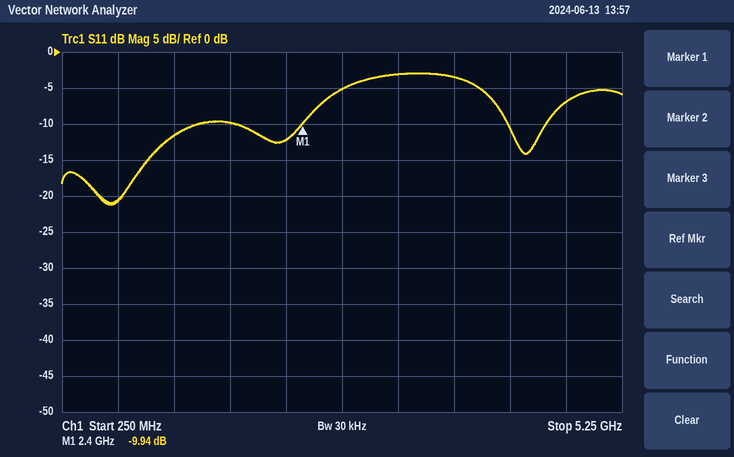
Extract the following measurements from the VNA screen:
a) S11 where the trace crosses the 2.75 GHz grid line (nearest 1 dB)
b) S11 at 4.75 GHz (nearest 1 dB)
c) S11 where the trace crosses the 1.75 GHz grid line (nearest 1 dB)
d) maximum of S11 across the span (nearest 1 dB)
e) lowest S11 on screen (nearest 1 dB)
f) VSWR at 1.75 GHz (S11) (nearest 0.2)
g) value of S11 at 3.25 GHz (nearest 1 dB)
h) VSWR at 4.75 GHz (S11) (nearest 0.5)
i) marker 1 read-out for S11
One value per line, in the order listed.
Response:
-5 dB
-7 dB
-10 dB
-3 dB
-21 dB
2.0
-3 dB
2.5
-9.94 dB
